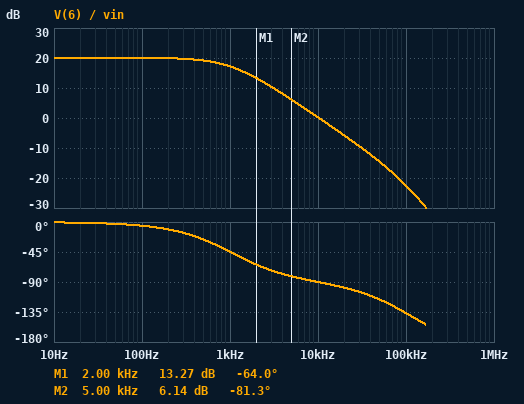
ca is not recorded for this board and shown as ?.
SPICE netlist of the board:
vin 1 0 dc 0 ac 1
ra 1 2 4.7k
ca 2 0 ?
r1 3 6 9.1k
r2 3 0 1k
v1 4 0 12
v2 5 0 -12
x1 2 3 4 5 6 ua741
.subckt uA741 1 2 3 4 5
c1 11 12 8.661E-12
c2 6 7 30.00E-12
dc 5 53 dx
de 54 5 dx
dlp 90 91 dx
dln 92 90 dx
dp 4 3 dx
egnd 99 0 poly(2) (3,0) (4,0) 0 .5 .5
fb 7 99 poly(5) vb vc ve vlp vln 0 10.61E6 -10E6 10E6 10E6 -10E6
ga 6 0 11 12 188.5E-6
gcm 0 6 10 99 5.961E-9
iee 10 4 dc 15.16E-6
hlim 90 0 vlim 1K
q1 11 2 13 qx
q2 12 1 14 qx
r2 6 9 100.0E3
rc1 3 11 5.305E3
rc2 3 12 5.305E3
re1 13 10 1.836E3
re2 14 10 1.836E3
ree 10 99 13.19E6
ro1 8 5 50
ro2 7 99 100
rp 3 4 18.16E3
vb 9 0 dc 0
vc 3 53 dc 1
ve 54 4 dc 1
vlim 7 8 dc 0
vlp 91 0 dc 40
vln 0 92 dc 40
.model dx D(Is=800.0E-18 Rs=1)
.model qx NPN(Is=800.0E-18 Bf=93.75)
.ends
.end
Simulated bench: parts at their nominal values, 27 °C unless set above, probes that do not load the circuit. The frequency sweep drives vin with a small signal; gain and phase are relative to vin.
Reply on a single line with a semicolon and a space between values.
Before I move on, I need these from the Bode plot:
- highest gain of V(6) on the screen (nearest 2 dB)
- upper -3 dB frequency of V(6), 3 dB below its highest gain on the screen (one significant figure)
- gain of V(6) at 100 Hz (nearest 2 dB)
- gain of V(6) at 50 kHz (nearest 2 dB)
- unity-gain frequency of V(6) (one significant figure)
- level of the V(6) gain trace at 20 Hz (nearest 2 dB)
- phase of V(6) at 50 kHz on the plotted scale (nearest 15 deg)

20 dB; 1 kHz; 20 dB; -14 dB; 10 kHz; 20 dB; -120 deg
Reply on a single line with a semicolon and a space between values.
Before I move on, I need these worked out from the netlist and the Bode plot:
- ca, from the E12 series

33 nF
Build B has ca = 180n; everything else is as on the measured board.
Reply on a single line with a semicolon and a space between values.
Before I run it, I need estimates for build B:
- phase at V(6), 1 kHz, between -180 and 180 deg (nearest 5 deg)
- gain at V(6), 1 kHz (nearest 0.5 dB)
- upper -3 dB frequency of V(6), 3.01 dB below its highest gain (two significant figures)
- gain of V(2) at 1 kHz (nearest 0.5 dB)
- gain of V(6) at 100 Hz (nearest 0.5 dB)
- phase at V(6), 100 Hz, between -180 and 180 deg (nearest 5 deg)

-80 deg; 5.5 dB; 190 Hz; -14.5 dB; 19.0 dB; -30 deg
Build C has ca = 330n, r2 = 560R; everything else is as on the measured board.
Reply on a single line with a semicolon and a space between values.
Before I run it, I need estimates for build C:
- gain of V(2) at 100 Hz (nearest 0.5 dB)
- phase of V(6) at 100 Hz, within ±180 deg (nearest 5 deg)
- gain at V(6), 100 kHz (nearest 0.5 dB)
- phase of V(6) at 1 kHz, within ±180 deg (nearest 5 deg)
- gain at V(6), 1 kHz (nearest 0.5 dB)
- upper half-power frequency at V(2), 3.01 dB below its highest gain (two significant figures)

-3.0 dB; -45 deg; -41.0 dB; -85 deg; 5.0 dB; 100 Hz
